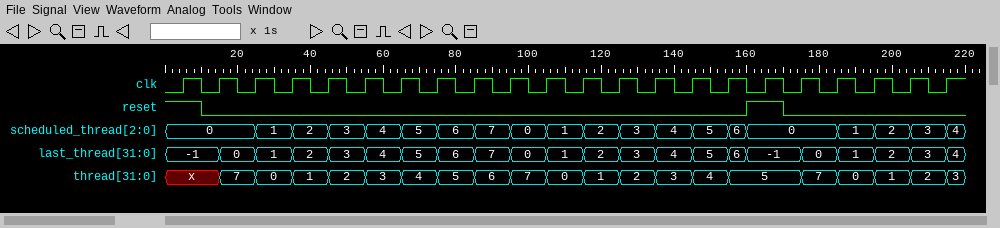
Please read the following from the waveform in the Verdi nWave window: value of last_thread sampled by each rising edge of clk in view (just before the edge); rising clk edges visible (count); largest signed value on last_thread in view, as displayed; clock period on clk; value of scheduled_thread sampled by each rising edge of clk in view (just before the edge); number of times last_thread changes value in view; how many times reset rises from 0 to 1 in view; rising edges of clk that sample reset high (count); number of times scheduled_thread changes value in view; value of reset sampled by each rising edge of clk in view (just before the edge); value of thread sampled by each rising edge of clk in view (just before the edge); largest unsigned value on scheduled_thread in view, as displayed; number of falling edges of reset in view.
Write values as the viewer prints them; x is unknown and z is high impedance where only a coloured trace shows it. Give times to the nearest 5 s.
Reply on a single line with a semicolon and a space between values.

-1, -1, 0, 1, 2, 3, 4, 5, 6, 7, 0, 1, 2, 3, 4, 5, -1, -1, 0, 1, 2, 3; 22; 7; 10 s; 0, 0, 0, 1, 2, 3, 4, 5, 6, 7, 0, 1, 2, 3, 4, 5, 0, 0, 0, 1, 2, 3; 21; 1; 2; 19; 1 0 0 0 0 0 0 0 0 0 0 0 0 0 0 0 1 0 0 0 0 0; x, x, 7, 0, 1, 2, 3, 4, 5, 6, 7, 0, 1, 2, 3, 4, 5, 5, 7, 0, 1, 2; 7; 2
